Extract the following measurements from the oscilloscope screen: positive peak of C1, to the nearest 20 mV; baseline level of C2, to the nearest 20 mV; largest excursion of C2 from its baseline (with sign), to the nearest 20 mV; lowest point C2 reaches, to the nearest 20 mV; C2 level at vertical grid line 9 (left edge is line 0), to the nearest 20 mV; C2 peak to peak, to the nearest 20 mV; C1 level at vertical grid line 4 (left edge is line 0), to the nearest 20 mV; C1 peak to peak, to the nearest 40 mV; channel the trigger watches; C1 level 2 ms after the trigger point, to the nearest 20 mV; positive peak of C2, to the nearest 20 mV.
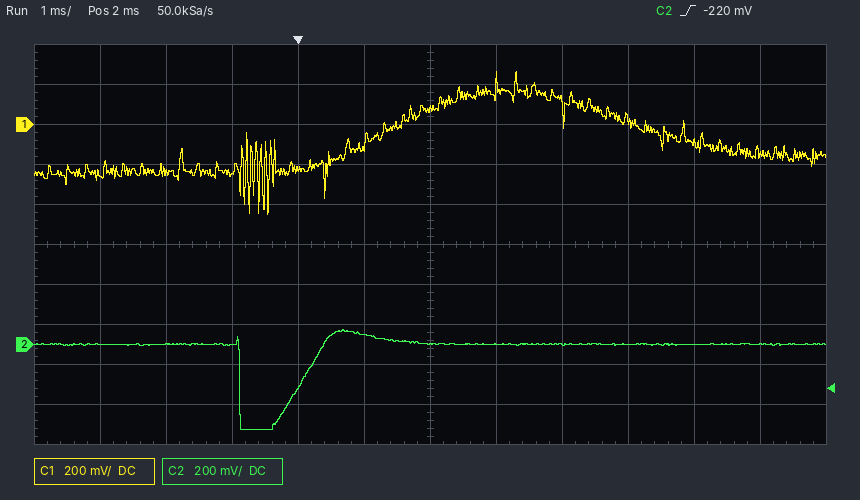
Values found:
260 mV
0 mV
-420 mV
-420 mV
0 mV
500 mV
-220 mV
720 mV
C2
80 mV
80 mV
